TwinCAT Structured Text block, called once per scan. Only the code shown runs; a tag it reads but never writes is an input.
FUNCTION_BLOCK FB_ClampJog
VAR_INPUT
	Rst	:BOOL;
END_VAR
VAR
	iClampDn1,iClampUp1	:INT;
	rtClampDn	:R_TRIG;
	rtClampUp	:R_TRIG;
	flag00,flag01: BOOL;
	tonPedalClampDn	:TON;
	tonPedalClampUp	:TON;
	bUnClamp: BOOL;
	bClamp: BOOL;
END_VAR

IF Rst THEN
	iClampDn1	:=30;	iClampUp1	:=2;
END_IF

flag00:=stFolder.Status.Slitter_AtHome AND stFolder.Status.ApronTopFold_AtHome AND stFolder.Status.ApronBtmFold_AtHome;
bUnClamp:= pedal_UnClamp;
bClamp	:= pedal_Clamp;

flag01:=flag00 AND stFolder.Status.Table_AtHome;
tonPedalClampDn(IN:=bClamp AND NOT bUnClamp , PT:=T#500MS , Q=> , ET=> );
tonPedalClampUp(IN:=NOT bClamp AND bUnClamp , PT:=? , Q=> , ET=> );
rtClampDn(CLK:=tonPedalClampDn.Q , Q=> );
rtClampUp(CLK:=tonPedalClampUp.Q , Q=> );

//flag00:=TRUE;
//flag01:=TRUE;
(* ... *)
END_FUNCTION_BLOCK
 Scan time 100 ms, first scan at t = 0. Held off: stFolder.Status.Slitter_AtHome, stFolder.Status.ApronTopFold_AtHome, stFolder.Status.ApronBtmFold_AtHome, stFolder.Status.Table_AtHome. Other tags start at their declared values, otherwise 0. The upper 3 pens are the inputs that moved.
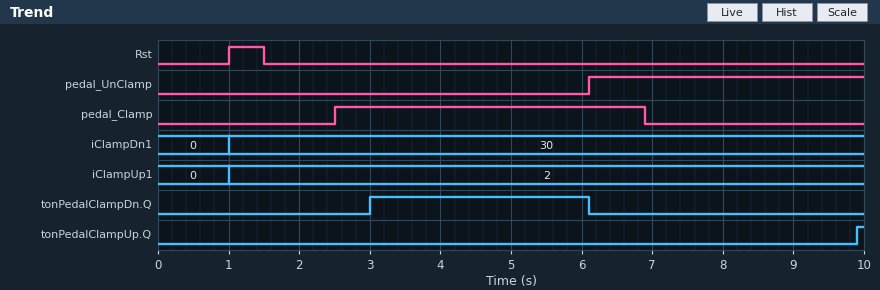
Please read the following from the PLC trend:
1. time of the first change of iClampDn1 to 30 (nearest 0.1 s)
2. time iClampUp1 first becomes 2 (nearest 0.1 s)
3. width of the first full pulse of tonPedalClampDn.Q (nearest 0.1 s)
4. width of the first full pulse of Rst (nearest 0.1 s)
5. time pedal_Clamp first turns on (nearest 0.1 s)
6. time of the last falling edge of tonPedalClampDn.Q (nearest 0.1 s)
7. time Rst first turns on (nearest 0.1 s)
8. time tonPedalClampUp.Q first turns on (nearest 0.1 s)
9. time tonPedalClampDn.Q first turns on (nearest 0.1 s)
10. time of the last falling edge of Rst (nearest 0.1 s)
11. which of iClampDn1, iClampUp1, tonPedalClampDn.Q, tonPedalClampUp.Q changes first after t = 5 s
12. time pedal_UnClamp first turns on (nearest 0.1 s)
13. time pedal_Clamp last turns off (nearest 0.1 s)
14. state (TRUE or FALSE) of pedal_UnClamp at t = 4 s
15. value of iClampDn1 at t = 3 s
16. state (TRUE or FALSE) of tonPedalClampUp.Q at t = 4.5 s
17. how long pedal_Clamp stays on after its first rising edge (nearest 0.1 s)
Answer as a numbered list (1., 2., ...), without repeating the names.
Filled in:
1. 1.0 s
2. 1.0 s
3. 3.1 s
4. 0.5 s
5. 2.5 s
6. 6.1 s
7. 1.0 s
8. 9.9 s
9. 3.0 s
10. 1.5 s
11. tonPedalClampDn.Q
12. 6.1 s
13. 6.9 s
14. FALSE
15. 30
16. FALSE
17. 4.4 s
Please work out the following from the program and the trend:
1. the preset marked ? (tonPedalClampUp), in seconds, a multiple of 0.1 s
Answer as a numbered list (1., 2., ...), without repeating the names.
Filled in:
1. 3.0 s
